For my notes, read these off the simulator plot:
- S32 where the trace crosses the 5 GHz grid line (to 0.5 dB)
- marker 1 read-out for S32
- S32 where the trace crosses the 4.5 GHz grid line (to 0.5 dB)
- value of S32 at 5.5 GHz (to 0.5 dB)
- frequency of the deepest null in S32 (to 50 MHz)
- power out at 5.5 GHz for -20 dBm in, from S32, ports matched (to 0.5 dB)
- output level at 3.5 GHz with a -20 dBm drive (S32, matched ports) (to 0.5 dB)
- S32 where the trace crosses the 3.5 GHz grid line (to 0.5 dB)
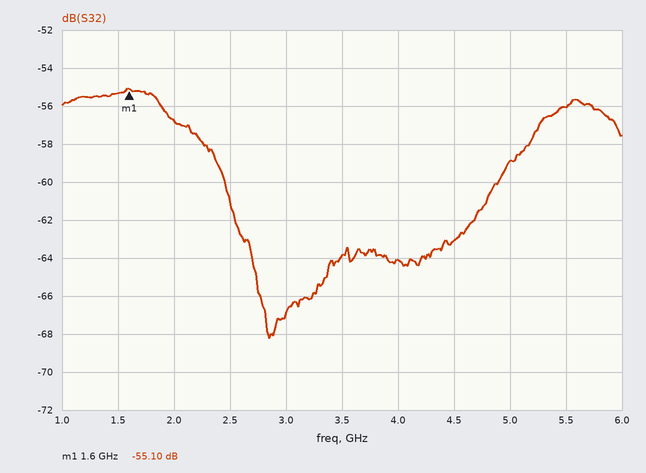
-59.0 dB
-55.10 dB
-63.0 dB
-56.0 dB
2.85 GHz
-76.0 dBm
-84.0 dBm
-64.0 dB
